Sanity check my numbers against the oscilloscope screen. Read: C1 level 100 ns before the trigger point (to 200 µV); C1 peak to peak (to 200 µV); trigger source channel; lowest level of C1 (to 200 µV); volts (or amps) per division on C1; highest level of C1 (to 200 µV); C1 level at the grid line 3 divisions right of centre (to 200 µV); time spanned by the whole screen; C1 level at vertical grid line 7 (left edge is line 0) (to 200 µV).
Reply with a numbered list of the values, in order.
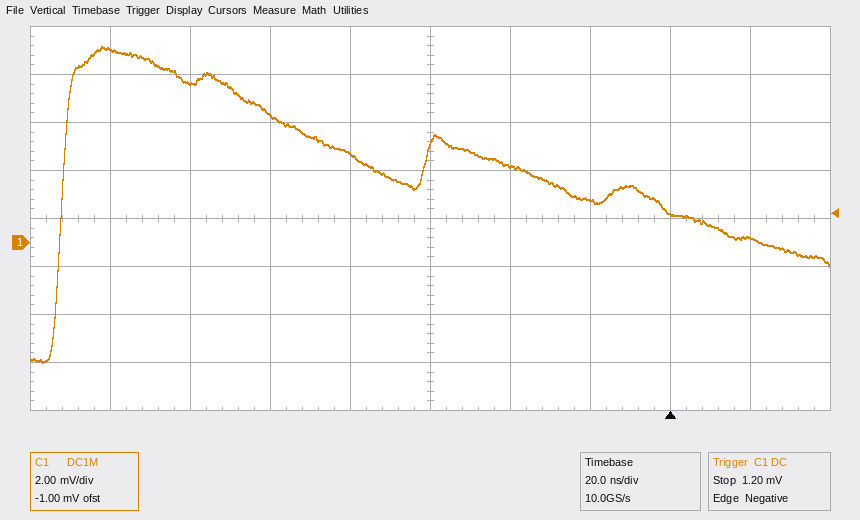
1. 5.4 mV
2. 13.2 mV
3. C1
4. -5.0 mV
5. 2 mV
6. 8.2 mV
7. 1.2 mV
8. 200 ns
9. 1.8 mV
